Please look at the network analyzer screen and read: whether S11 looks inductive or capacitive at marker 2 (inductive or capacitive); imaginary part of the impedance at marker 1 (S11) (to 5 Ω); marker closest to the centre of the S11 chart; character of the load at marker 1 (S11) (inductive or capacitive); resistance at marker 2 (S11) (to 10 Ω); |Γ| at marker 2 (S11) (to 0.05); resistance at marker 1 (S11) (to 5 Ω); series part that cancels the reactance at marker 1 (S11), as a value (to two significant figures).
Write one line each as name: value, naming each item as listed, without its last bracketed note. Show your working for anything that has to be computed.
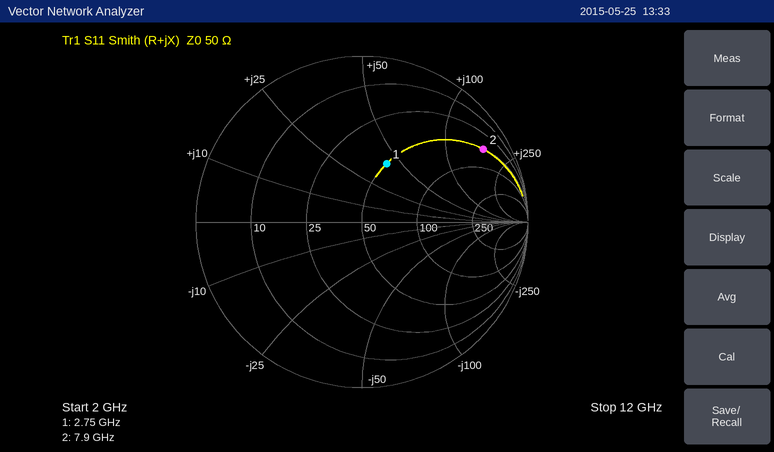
whether S11 looks inductive or capacitive at marker 2: inductive
imaginary part of the impedance at marker 1 (S11): +40 Ω
marker closest to the centre of the S11 chart: marker 1
character of the load at marker 1 (S11): inductive
resistance at marker 2 (S11): 50 Ω
|Γ| at marker 2 (S11): 0.85
resistance at marker 1 (S11): 50 Ω
series part that cancels the reactance at marker 1 (S11), as a value: C = 1/(2π × 2.75 GHz × 40 Ω) ≈ 1.4 pF
